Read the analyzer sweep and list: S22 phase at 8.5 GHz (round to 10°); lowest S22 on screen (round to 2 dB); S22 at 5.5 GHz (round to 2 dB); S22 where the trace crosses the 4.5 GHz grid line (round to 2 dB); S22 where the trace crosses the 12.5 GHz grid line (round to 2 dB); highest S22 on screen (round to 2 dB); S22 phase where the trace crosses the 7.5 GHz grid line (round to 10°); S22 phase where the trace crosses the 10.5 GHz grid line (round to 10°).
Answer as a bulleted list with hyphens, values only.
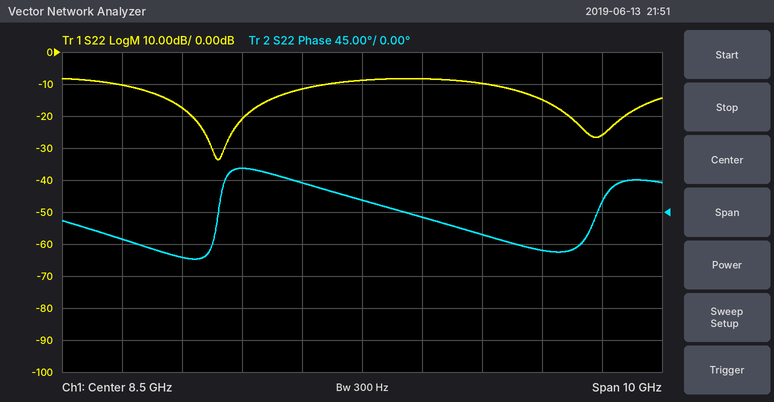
- 20°
- -34 dB
- -18 dB
- -10 dB
- -26 dB
- -8 dB
- 40°
- -30°
